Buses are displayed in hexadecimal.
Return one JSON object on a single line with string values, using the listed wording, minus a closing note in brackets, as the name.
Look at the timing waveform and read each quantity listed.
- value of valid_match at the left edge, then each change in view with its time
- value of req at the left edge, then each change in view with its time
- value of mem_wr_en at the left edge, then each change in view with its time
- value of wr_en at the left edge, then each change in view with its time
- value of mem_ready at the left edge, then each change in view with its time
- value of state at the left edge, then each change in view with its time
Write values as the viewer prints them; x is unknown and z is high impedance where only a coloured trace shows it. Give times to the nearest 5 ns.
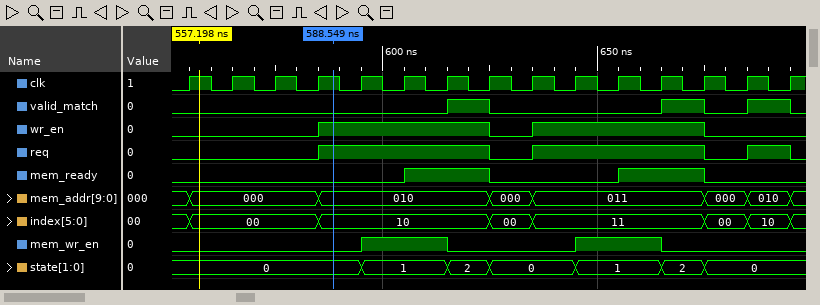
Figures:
{"value of valid_match at the left edge, then each change in view with its time": "0, 1 at 615 ns, 0 at 625 ns, 1 at 665 ns, 0 at 675 ns, 1 at 685 ns, 0 at 695 ns", "value of req at the left edge, then each change in view with its time": "0, 1 at 585 ns, 0 at 625 ns, 1 at 635 ns, 0 at 675 ns, 1 at 685 ns, 0 at 695 ns", "value of mem_wr_en at the left edge, then each change in view with its time": "0, 1 at 595 ns, 0 at 615 ns, 1 at 645 ns, 0 at 665 ns", "value of wr_en at the left edge, then each change in view with its time": "0, 1 at 585 ns, 0 at 625 ns, 1 at 635 ns, 0 at 675 ns", "value of mem_ready at the left edge, then each change in view with its time": "0, 1 at 605 ns, 0 at 625 ns, 1 at 655 ns, 0 at 675 ns", "value of state at the left edge, then each change in view with its time": "0, 1 at 595 ns, 2 at 615 ns, 0 at 625 ns, 1 at 645 ns, 2 at 665 ns, 0 at 675 ns"}
